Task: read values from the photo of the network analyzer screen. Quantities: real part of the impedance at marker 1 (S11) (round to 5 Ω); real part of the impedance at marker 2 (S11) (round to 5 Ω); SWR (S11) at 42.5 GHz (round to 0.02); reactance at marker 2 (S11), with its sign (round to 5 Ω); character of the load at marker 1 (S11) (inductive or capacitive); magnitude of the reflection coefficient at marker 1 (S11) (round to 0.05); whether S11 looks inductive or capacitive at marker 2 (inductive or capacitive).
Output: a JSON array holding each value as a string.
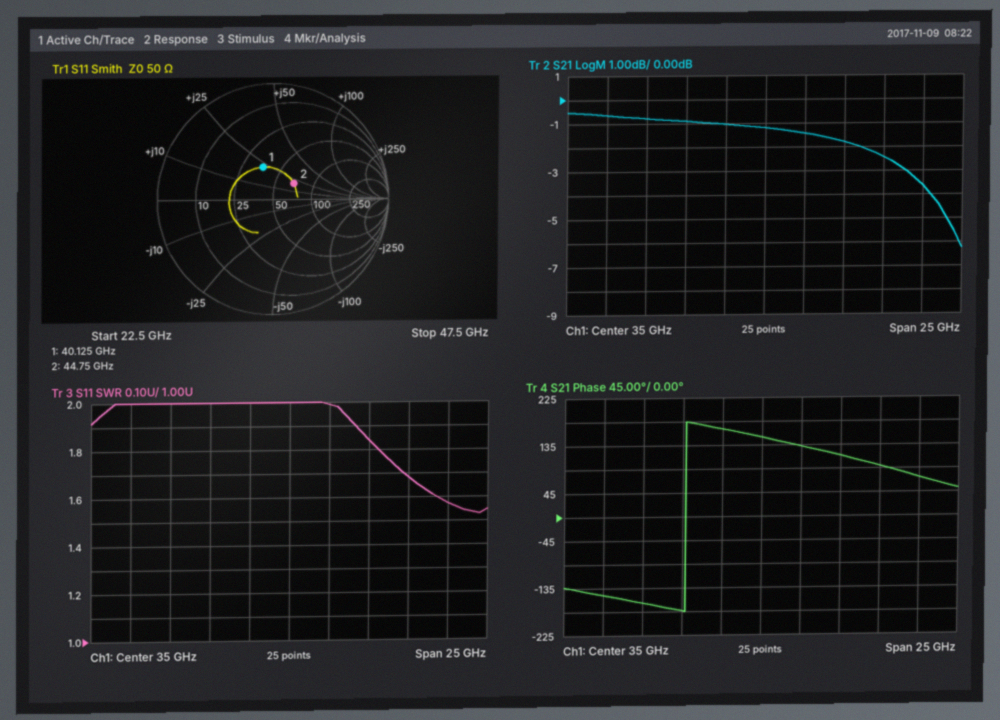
["35 Ω", "70 Ω", "1.68", "+20 Ω", "inductive", "0.30", "inductive"]
